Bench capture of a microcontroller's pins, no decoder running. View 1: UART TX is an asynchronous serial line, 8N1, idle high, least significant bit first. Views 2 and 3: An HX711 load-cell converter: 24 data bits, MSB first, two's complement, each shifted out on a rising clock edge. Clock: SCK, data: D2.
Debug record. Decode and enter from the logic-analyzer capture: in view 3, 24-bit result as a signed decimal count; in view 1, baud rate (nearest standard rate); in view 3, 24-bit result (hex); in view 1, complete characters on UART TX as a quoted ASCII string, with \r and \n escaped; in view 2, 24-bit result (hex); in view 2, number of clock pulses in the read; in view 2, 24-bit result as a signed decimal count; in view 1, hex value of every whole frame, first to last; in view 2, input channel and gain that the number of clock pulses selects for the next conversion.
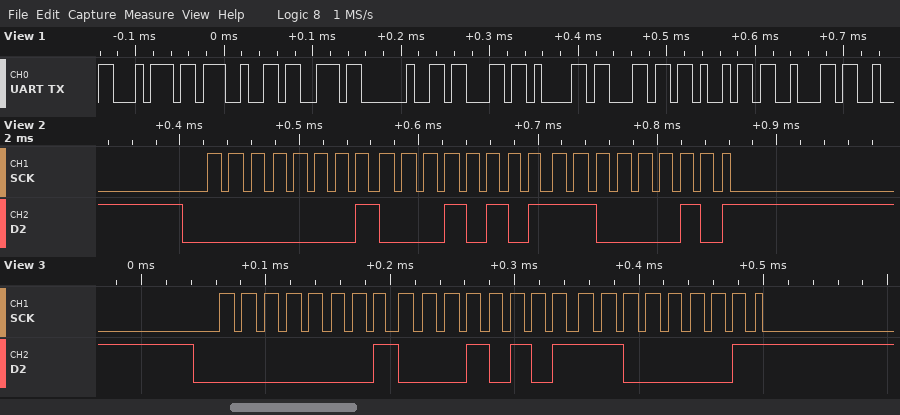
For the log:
71105
115200 baud
0x0115C1
"t's calib"
0x0115C2
25
71106
0x74 0x27 0x73 0x20 0x63 0x61 0x6C 0x69 0x62
channel A, gain 128
